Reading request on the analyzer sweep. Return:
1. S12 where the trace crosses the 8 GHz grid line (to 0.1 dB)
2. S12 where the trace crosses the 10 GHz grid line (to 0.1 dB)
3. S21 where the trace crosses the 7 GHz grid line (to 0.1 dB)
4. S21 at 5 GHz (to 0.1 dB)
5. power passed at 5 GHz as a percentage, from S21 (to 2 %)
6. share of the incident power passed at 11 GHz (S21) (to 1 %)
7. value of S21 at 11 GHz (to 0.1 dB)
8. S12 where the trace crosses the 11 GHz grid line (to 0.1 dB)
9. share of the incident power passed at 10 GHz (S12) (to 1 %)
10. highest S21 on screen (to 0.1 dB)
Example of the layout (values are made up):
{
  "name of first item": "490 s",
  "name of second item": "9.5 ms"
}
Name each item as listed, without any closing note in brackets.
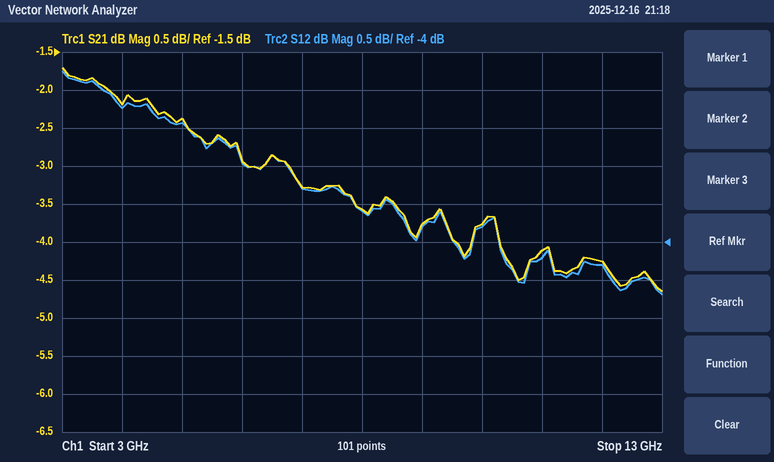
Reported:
{
  "S12 where the trace crosses the 8 GHz grid line": "-3.6 dB",
  "S12 where the trace crosses the 10 GHz grid line": "-3.8 dB",
  "S21 where the trace crosses the 7 GHz grid line": "-3.3 dB",
  "S21 at 5 GHz": "-2.4 dB",
  "power passed at 5 GHz as a percentage, from S21": "58 %",
  "share of the incident power passed at 11 GHz (S21)": "39 %",
  "value of S21 at 11 GHz": "-4.1 dB",
  "S12 where the trace crosses the 11 GHz grid line": "-4.2 dB",
  "share of the incident power passed at 10 GHz (S12)": "42 %",
  "highest S21 on screen": "-1.7 dB"
}
